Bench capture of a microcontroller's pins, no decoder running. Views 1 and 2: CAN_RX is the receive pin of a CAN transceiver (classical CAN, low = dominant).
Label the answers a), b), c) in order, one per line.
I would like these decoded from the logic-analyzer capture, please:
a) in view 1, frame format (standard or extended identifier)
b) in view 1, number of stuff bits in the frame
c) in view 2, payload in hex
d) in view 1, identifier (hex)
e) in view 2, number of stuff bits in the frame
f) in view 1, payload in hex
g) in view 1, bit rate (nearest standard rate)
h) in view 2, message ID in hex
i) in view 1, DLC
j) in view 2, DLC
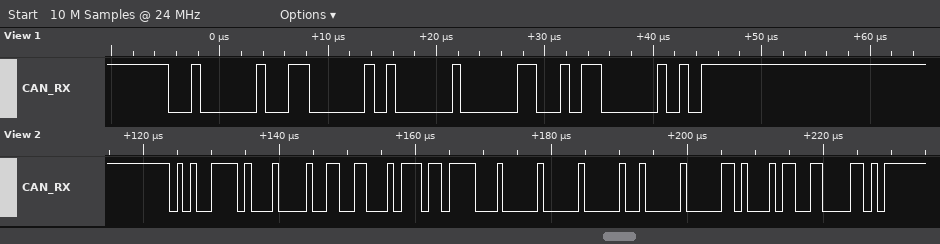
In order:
a) standard
b) 5
c) 4C C5 DB C4 00 01 00 28
d) 0x203
e) 5
f) 00
g) 1000 kbit/s
h) 0x53D
i) 1
j) 8
